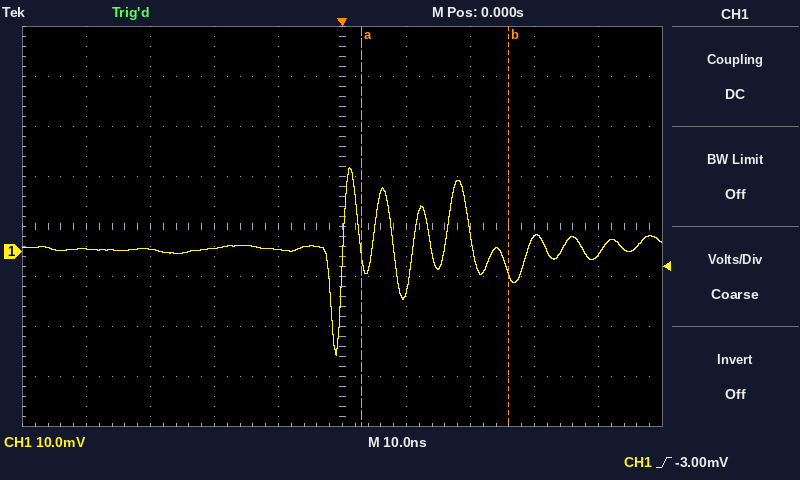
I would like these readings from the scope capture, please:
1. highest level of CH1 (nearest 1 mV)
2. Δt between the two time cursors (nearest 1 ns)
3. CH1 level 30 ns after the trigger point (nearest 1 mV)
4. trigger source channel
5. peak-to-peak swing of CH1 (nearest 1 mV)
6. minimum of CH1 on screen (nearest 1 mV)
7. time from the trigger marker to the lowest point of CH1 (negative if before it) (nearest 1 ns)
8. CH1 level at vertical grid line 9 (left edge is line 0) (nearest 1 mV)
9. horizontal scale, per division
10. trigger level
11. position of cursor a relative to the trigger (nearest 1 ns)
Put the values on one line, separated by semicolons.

17 mV; 23 ns; 3 mV; CH1; 38 mV; -21 mV; -1 ns; -1 mV; 10 ns; -3.00 mV; +3 ns
